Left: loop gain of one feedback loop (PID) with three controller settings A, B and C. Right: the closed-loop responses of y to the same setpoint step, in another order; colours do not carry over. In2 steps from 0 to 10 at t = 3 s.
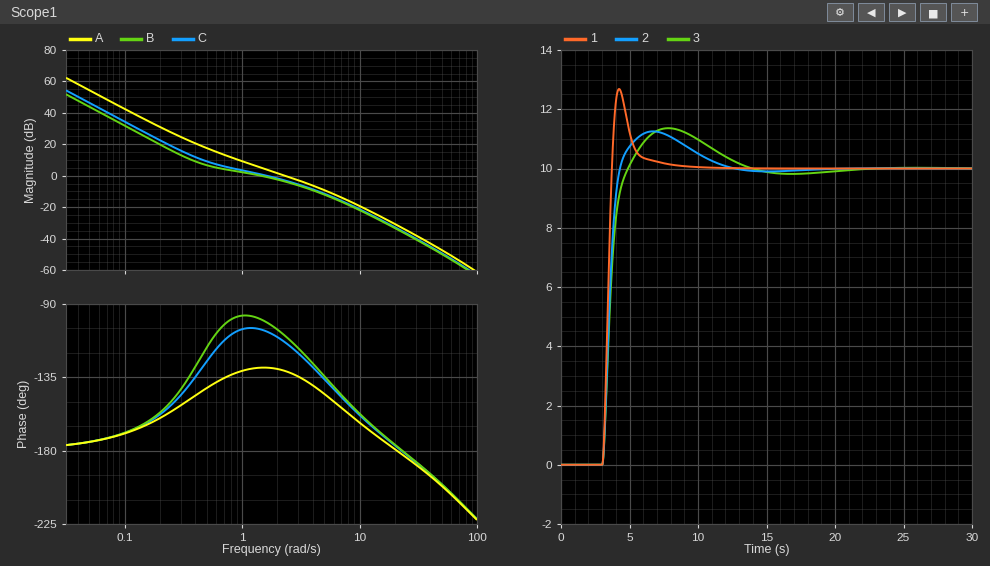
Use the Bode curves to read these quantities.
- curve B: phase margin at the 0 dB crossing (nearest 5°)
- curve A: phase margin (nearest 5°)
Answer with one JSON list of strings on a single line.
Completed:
["80°", "50°"]
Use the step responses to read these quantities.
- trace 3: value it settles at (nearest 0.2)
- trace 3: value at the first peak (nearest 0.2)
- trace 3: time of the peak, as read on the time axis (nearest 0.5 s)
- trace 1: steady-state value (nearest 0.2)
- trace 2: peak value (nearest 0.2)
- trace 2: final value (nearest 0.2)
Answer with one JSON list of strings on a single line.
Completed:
["10.0", "11.4", "8.0 s", "10.0", "11.2", "10.0"]
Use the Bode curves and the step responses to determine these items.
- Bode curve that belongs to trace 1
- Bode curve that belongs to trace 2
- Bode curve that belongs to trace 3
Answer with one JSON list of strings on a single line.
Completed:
["A", "C", "B"]
